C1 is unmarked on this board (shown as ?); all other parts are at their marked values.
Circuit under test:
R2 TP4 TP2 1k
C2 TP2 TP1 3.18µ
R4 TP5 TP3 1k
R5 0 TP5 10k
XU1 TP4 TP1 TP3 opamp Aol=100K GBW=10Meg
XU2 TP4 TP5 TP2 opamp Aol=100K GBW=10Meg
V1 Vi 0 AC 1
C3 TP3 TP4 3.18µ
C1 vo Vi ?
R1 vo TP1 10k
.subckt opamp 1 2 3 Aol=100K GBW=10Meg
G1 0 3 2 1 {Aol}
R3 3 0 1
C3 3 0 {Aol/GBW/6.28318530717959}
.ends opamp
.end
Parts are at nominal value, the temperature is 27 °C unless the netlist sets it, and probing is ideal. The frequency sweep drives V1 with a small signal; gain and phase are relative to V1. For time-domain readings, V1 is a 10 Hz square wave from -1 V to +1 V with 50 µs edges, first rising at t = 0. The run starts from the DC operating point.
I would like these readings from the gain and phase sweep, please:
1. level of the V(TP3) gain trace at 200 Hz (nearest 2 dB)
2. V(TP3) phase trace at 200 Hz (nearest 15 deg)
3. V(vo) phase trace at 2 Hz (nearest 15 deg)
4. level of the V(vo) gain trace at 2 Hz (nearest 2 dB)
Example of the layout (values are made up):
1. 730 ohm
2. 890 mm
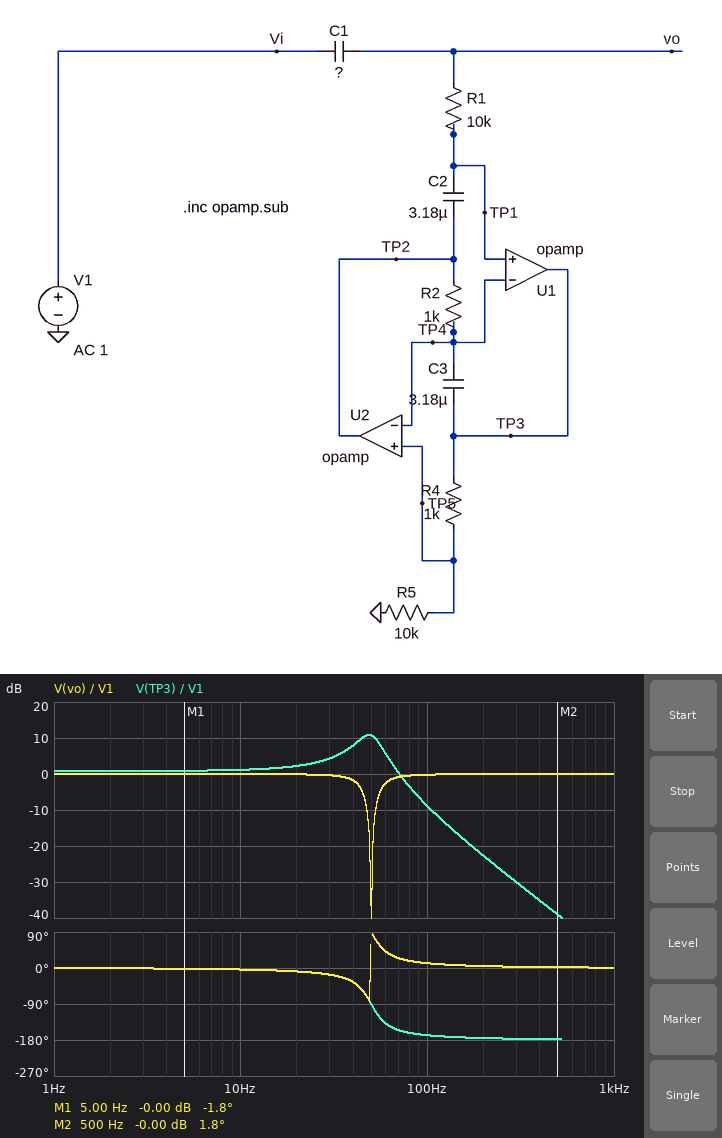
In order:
1. -22 dB
2. -180 deg
3. 0 deg
4. 0 dB
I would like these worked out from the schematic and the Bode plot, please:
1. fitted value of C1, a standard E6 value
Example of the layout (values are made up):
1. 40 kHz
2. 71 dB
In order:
1. 1 µF
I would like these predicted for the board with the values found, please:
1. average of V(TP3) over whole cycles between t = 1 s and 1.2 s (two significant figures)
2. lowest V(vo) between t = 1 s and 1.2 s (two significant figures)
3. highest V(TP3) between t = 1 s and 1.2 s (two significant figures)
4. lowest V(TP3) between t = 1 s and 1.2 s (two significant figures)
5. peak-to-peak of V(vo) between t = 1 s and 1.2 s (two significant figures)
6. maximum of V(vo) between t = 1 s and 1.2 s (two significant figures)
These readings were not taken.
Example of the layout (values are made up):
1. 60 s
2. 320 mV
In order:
1. 1.1 V
2. -330 mV
3. 3.6 V
4. -1.4 V
5. 2.7 V
6. 2.3 V
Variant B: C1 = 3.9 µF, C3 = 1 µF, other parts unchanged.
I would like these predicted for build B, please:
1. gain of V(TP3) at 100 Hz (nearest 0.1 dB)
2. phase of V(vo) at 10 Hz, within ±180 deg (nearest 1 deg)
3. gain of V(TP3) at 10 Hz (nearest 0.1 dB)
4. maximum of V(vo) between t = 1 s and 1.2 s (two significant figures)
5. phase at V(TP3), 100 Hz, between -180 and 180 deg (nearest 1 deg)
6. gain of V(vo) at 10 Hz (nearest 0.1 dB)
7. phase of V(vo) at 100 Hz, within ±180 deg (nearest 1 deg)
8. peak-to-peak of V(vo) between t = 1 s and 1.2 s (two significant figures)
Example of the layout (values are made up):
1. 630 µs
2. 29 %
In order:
1. 12.5 dB
2. 0 deg
3. 0.9 dB
4. 2.2 V
5. -169 deg
6. 0 dB
7. 11 deg
8. 2.3 V
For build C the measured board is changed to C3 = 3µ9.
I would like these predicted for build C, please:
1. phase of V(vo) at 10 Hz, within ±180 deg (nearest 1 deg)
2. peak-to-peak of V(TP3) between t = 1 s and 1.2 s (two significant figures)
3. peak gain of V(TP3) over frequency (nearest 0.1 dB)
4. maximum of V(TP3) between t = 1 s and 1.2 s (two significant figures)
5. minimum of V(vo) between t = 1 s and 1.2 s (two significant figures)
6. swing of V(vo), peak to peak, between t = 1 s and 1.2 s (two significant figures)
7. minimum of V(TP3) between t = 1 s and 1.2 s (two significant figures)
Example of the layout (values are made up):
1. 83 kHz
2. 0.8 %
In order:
1. -5 deg
2. 4.6 V
3. 10.0 dB
4. 3.4 V
5. -300 mV
6. 2.6 V
7. -1.2 V
